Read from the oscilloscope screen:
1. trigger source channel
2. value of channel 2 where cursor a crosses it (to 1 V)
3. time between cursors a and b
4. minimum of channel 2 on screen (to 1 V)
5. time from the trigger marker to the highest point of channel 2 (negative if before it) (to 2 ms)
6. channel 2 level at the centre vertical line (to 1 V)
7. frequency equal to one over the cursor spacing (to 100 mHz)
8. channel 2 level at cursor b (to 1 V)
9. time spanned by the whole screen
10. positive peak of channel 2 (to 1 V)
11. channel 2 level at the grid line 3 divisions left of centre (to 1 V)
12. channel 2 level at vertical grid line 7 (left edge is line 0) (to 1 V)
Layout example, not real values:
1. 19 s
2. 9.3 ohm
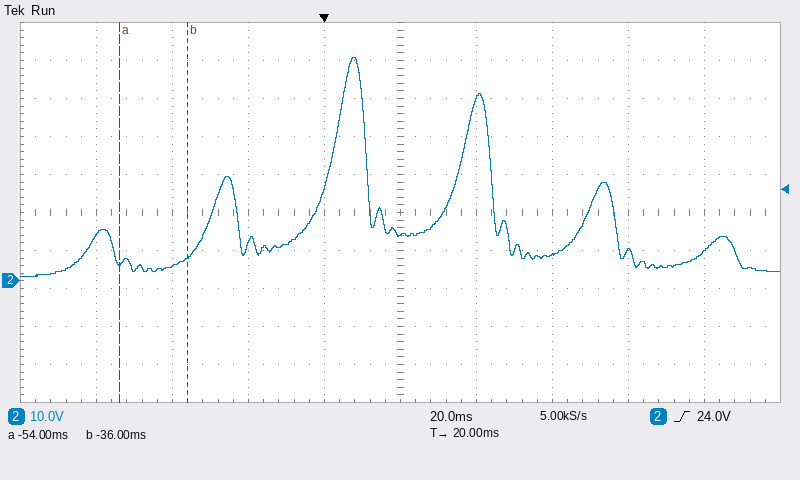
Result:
1. channel 2
2. 5 V
3. 18 ms
4. 1 V
5. +8 ms
6. 12 V
7. 55.6 Hz
8. 6 V
9. 200 ms
10. 59 V
11. 4 V
12. 7 V
